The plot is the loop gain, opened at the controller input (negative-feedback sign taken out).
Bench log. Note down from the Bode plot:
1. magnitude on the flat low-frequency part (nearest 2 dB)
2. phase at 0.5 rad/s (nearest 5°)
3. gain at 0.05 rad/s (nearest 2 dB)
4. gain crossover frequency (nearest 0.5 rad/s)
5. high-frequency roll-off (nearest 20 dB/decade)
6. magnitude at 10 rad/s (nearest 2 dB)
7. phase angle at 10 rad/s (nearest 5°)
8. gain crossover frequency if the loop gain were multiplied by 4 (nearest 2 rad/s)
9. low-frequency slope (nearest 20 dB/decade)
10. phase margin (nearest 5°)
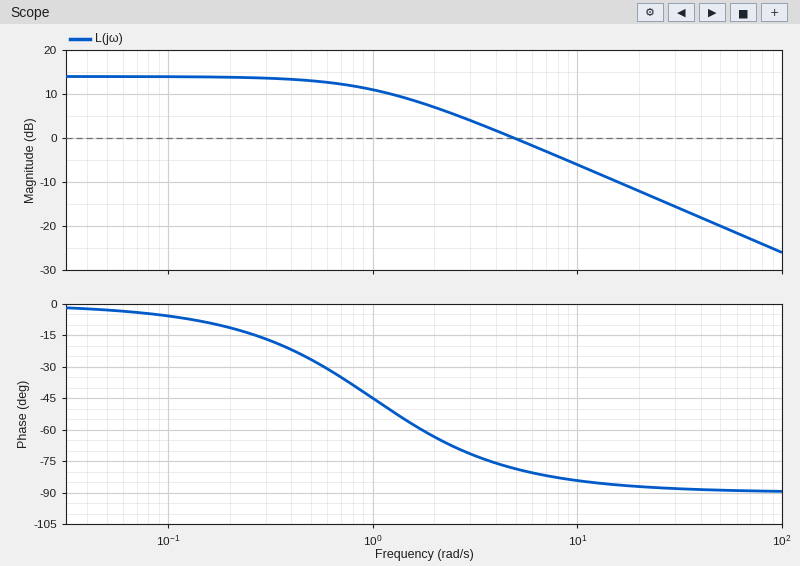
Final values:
14 dB
-25°
14 dB
5.0 rad/s
-20 dB/decade
-6 dB
-85°
20 rad/s
0 dB/decade
100°
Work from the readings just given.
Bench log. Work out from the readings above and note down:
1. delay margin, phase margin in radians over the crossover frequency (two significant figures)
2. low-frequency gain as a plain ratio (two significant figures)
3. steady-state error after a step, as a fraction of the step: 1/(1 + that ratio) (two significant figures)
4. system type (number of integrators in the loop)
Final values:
0.35 s
5.0
0.17
0
